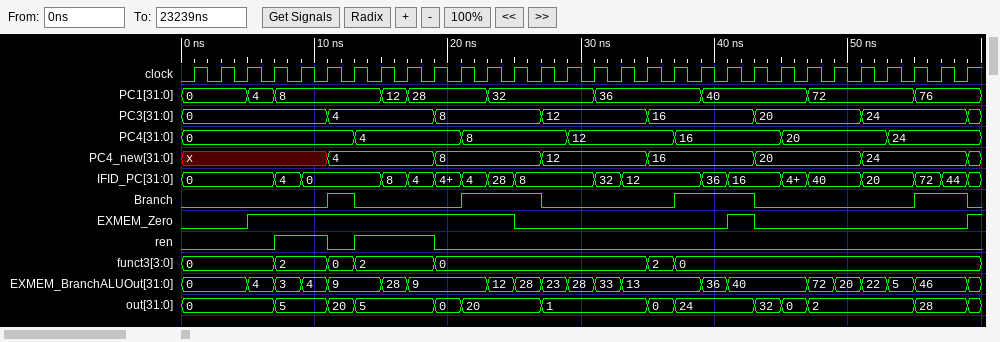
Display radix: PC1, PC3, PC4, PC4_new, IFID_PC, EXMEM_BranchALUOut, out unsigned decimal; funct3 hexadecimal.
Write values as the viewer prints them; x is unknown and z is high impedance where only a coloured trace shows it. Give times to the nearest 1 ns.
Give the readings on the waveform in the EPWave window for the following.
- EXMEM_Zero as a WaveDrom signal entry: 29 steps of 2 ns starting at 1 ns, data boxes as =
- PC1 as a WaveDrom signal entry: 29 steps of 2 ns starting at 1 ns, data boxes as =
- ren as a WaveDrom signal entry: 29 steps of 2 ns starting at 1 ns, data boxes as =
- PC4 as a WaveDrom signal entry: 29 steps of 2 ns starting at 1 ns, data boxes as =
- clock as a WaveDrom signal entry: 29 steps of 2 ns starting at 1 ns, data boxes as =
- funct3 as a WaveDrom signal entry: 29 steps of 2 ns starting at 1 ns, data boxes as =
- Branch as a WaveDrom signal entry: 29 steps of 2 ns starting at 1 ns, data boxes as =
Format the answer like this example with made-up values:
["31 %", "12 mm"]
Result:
["{name: 'EXMEM_Zero', wave: '0.1.........0.......10.......'}", "{name: 'PC1', wave: '=.==...==..=...=...=...=...=.', data: '0 4 8 12 28 32 36 40 72 76'}", "{name: 'ren', wave: '0..1.01..0...................'}", "{name: 'PC4', wave: '=.....=...=...=...=...=...=..', data: '0 4 8 12 16 20 24'}", "{name: 'clock', wave: 'p............................'}", "{name: 'funct3', wave: '=..=.==..=.......==..........', data: '0 2 0 2 0 2 0'}", "{name: 'Branch', wave: '0....10...1..0....1..0.....1.'}"]
